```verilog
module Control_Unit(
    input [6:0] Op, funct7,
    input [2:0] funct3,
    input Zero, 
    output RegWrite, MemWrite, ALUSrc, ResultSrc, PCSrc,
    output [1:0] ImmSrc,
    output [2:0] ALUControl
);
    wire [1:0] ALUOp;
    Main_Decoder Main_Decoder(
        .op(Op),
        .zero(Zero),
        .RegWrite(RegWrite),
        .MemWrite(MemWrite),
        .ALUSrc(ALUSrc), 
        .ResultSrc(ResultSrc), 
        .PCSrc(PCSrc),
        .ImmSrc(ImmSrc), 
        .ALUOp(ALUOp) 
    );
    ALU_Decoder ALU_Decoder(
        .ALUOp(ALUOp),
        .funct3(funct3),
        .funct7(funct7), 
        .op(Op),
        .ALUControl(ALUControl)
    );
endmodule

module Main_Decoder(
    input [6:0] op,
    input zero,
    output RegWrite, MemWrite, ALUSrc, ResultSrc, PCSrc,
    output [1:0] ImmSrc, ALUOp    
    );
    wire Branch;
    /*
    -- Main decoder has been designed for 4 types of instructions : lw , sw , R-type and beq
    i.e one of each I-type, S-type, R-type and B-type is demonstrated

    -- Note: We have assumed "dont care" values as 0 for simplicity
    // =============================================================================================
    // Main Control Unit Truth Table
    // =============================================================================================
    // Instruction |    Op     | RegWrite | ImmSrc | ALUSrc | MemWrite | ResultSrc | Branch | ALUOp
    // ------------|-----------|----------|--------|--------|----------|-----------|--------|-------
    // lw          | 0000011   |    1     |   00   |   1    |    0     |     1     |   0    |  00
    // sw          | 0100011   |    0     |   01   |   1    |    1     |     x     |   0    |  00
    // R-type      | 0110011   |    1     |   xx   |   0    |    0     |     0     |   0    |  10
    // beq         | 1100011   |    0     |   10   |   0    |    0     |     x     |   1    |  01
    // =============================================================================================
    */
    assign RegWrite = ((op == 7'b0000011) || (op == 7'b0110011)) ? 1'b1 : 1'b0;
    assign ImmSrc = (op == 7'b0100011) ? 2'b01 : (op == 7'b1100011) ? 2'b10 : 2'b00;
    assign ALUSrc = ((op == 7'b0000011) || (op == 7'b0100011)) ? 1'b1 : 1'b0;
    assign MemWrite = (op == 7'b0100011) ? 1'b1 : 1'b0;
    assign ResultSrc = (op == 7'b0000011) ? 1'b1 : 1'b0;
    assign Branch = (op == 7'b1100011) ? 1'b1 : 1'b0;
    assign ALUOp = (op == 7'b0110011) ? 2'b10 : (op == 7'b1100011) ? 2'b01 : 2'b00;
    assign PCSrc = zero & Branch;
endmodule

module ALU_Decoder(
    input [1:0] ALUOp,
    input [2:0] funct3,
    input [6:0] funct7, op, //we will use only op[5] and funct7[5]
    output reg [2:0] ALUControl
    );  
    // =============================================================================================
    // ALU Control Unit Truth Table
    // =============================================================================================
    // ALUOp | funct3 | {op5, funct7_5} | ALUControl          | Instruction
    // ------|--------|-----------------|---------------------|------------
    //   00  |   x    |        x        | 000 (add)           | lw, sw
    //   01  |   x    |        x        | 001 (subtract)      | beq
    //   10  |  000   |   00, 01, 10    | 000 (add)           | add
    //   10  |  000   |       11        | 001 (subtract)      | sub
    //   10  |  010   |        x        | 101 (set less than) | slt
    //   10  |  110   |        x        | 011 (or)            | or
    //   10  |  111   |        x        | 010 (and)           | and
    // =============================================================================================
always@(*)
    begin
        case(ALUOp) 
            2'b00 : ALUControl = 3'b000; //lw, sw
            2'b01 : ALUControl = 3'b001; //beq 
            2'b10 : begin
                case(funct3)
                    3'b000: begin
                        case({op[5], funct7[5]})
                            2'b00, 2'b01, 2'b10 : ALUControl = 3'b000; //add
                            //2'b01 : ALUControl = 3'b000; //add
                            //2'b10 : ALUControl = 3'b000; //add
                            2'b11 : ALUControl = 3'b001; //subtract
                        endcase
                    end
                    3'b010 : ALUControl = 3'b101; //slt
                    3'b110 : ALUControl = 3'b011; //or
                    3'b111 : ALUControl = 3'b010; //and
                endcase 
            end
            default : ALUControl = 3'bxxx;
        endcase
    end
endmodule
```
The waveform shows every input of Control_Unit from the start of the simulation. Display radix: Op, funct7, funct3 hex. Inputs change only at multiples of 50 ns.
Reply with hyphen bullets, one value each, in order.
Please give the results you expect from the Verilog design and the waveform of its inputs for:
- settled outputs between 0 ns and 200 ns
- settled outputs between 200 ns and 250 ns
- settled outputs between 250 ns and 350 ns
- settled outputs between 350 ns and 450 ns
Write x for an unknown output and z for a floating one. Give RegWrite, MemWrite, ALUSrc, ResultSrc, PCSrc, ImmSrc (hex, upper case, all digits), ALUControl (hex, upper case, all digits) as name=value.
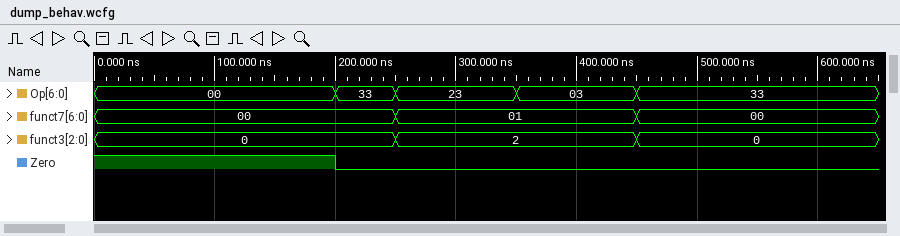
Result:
- RegWrite=0, MemWrite=0, ALUSrc=0, ResultSrc=0, PCSrc=0, ImmSrc=0, ALUControl=0
- RegWrite=1, MemWrite=0, ALUSrc=0, ResultSrc=0, PCSrc=0, ImmSrc=0, ALUControl=0
- RegWrite=0, MemWrite=1, ALUSrc=1, ResultSrc=0, PCSrc=0, ImmSrc=1, ALUControl=0
- RegWrite=1, MemWrite=0, ALUSrc=1, ResultSrc=1, PCSrc=0, ImmSrc=0, ALUControl=0
